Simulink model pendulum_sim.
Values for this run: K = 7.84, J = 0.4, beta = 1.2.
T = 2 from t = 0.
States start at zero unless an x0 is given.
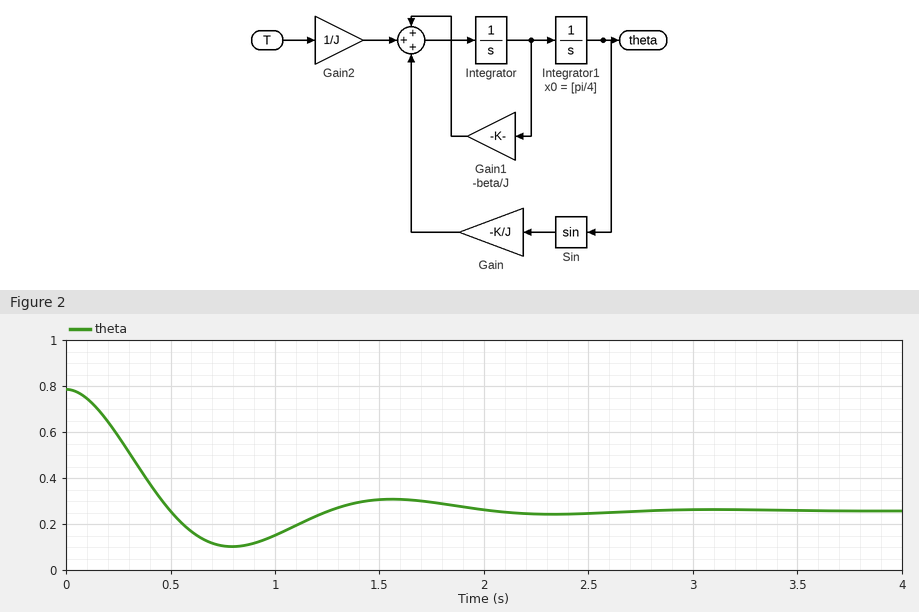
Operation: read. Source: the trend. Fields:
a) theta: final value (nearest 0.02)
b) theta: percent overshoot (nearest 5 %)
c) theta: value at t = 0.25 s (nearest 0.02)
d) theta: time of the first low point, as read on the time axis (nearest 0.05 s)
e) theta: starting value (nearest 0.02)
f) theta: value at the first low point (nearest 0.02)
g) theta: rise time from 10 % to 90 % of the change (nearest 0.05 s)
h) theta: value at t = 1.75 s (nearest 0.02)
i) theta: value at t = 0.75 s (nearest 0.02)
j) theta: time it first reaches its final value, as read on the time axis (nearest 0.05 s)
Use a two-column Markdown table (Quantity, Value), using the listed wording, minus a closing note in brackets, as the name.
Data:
| Quantity | Value |
|---|---|
| theta: final value | 0.26 |
| theta: percent overshoot | 30 % |
| theta: value at t = 0.25 s | 0.58 |
| theta: time of the first low point, as read on the time axis | 0.80 s |
| theta: starting value | 0.78 |
| theta: value at the first low point | 0.10 |
| theta: rise time from 10 % to 90 % of the change | 0.35 s |
| theta: value at t = 1.75 s | 0.30 |
| theta: value at t = 0.75 s | 0.10 |
| theta: time it first reaches its final value, as read on the time axis | 0.50 s |
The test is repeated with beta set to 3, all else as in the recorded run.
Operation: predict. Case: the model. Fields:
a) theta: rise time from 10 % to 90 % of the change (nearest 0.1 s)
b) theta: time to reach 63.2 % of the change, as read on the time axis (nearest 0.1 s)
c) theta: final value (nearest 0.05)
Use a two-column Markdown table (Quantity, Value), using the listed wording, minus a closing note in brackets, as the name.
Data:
| Quantity | Value |
|---|---|
| theta: rise time from 10 % to 90 % of the change | 0.7 s |
| theta: time to reach 63.2 % of the change, as read on the time axis | 0.5 s |
| theta: final value | 0.25 |
